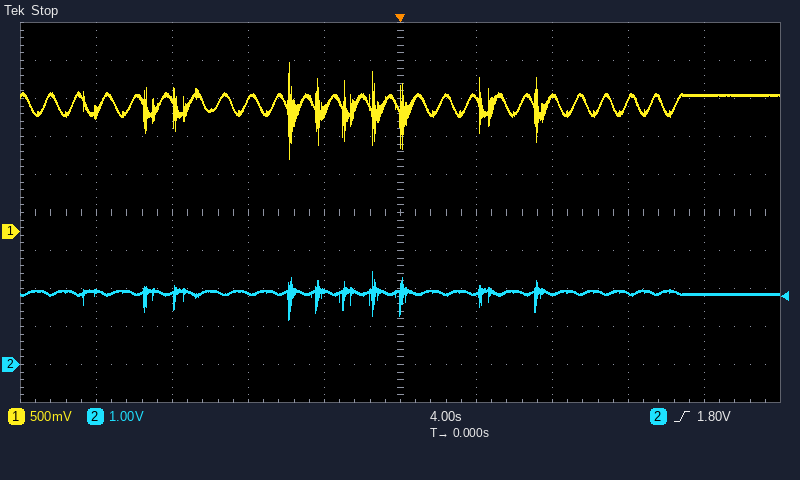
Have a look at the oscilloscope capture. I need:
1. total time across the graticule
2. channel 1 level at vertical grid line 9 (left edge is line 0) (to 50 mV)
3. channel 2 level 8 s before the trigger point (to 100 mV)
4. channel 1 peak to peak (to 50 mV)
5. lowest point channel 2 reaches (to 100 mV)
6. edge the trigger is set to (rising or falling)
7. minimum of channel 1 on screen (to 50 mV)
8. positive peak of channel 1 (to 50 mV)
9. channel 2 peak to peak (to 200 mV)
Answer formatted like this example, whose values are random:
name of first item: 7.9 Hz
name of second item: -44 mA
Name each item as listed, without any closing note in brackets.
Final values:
total time across the graticule: 40 s
channel 1 level at vertical grid line 9 (left edge is line 0): 1.80 V
channel 2 level 8 s before the trigger point: 1.9 V
channel 1 peak to peak: 1.25 V
lowest point channel 2 reaches: 1.2 V
edge the trigger is set to: rising
minimum of channel 1 on screen: 950 mV
positive peak of channel 1: 2.20 V
channel 2 peak to peak: 1.2 V
